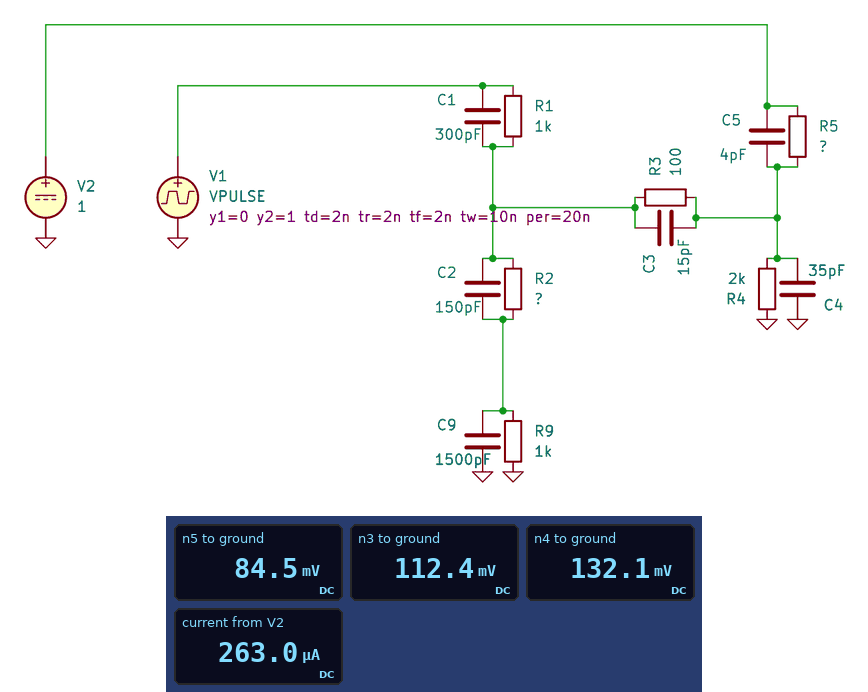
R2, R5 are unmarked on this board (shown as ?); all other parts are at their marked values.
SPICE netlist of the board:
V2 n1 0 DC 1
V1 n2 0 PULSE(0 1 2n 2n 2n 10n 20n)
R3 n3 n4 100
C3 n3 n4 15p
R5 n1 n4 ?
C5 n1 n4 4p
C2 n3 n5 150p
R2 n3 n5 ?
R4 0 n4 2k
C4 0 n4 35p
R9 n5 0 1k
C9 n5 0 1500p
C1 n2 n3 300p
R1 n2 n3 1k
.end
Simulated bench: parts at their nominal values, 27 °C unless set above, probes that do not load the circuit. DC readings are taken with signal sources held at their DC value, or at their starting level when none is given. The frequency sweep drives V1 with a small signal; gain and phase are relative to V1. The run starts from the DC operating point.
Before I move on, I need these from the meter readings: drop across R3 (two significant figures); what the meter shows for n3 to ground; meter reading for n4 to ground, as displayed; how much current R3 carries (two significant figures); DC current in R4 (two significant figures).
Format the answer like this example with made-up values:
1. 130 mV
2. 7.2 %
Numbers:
1. 20 mV
2. 112.4 mV
3. 132.1 mV
4. 200 µA
5. 66 µA
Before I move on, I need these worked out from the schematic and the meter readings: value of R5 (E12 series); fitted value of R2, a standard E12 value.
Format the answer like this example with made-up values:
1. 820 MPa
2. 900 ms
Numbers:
1. 3.3 kΩ
2. 330 Ω
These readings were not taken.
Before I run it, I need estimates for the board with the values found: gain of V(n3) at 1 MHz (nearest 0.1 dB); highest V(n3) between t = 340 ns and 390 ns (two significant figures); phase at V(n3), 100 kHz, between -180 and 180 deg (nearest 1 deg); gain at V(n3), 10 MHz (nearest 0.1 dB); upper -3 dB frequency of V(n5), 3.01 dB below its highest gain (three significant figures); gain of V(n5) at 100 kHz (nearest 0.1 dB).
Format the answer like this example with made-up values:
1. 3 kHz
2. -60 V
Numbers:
1. -8.0 dB
2. 590 mV
3. -5 deg
4. -4.0 dB
5. 235 kHz
6. -11.2 dB
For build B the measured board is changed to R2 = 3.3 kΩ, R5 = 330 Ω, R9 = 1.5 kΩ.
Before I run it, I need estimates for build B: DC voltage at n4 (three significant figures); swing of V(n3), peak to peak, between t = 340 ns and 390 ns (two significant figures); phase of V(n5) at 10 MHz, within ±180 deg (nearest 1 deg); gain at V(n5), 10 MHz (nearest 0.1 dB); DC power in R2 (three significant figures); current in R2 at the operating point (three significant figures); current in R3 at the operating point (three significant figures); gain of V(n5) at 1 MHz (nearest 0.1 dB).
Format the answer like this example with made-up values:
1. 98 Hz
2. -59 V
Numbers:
1. 658 mV
2. 690 mV
3. 4 deg
4. -24.6 dB
5. 49.3 µW
6. 122 µA
7. 709 µA
8. -27.5 dB
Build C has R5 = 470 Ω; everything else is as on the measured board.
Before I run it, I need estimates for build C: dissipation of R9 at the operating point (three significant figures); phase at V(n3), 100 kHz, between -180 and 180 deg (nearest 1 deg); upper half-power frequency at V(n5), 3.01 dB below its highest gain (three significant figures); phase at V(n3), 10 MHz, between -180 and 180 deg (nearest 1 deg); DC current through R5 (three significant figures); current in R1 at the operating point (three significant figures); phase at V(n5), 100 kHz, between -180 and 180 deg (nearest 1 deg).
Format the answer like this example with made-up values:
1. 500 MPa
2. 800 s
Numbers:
1. 109 µW
2. 0 deg
3. 325 kHz
4. 8 deg
5. 1.03 mA
6. 440 µA
7. -12 deg
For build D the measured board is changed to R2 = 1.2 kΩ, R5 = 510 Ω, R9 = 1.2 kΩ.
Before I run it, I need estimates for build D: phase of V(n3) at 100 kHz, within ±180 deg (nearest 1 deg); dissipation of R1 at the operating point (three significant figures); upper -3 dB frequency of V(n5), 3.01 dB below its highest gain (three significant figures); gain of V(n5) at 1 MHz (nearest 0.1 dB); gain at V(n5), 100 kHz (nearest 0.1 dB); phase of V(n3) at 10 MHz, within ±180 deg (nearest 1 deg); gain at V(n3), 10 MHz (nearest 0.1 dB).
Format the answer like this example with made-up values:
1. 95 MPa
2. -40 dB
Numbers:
1. 4 deg
2. 215 µW
3. 163 kHz
4. -25.3 dB
5. -18.1 dB
6. 5 deg
7. -3.8 dB
